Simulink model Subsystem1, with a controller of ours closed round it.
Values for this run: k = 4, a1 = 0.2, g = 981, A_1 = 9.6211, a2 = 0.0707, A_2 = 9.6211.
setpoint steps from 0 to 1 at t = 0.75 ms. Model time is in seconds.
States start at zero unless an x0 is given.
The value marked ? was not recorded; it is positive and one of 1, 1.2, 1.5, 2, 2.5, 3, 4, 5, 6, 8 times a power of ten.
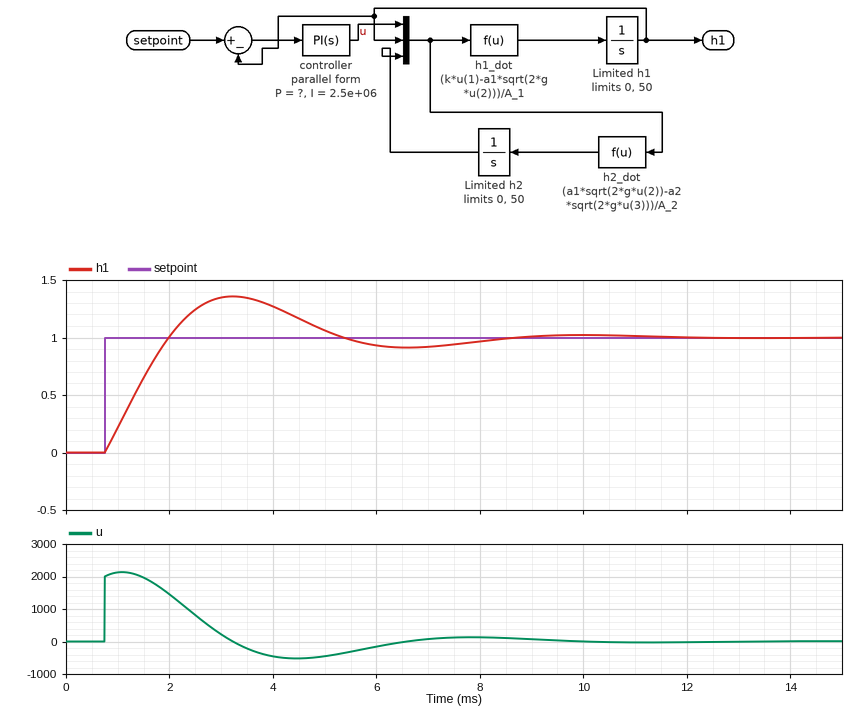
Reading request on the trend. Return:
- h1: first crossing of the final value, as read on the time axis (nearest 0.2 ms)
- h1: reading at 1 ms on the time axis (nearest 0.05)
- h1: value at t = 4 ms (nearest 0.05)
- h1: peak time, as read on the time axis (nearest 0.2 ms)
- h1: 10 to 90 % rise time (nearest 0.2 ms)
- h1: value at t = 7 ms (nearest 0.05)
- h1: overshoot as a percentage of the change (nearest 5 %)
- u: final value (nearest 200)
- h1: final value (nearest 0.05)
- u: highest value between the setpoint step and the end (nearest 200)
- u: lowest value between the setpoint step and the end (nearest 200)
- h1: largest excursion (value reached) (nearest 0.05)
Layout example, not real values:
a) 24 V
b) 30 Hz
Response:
a) 2.0 ms
b) 0.20
c) 1.25
d) 3.2 ms
e) 1.0 ms
f) 0.90
g) 35 %
h) 0
i) 1.00
j) 2200
k) -600
l) 1.35
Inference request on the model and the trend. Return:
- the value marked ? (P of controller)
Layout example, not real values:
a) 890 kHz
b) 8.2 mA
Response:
a) 2000
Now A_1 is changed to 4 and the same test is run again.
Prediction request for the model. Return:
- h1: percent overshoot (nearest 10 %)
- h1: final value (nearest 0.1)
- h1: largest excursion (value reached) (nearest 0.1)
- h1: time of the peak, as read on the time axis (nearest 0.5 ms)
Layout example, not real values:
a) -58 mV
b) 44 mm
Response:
a) 20 %
b) 1.0
c) 1.2
d) 2.0 ms
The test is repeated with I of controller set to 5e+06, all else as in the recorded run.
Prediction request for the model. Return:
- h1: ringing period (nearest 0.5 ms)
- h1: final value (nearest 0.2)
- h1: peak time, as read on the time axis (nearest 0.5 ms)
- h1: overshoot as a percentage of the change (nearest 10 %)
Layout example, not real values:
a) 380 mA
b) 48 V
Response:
a) 4.5 ms
b) 1.0
c) 2.5 ms
d) 50 %
